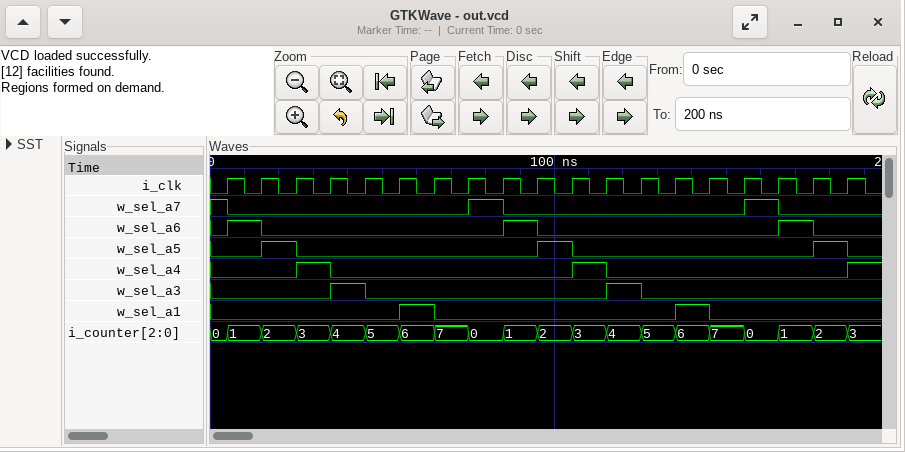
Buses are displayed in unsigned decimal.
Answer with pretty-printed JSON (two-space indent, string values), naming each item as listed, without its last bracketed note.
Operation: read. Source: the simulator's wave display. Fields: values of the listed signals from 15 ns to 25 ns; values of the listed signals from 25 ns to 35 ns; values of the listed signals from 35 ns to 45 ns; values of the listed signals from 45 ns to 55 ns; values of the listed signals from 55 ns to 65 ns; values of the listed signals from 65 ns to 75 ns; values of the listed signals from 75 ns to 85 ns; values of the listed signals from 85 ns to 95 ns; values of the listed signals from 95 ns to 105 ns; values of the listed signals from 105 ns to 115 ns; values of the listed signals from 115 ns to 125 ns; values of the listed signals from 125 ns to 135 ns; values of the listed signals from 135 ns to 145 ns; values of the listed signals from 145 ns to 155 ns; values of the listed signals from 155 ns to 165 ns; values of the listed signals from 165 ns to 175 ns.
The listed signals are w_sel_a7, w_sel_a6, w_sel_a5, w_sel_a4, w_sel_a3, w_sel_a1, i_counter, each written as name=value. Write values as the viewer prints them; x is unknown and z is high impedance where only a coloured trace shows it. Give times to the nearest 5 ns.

{
  "values of the listed signals from 15 ns to 25 ns": "w_sel_a7=0, w_sel_a6=0, w_sel_a5=1, w_sel_a4=0, w_sel_a3=0, w_sel_a1=0, i_counter=2",
  "values of the listed signals from 25 ns to 35 ns": "w_sel_a7=0, w_sel_a6=0, w_sel_a5=0, w_sel_a4=1, w_sel_a3=0, w_sel_a1=0, i_counter=3",
  "values of the listed signals from 35 ns to 45 ns": "w_sel_a7=0, w_sel_a6=0, w_sel_a5=0, w_sel_a4=0, w_sel_a3=1, w_sel_a1=0, i_counter=4",
  "values of the listed signals from 45 ns to 55 ns": "w_sel_a7=0, w_sel_a6=0, w_sel_a5=0, w_sel_a4=0, w_sel_a3=0, w_sel_a1=0, i_counter=5",
  "values of the listed signals from 55 ns to 65 ns": "w_sel_a7=0, w_sel_a6=0, w_sel_a5=0, w_sel_a4=0, w_sel_a3=0, w_sel_a1=1, i_counter=6",
  "values of the listed signals from 65 ns to 75 ns": "w_sel_a7=0, w_sel_a6=0, w_sel_a5=0, w_sel_a4=0, w_sel_a3=0, w_sel_a1=0, i_counter=7",
  "values of the listed signals from 75 ns to 85 ns": "w_sel_a7=1, w_sel_a6=0, w_sel_a5=0, w_sel_a4=0, w_sel_a3=0, w_sel_a1=0, i_counter=0",
  "values of the listed signals from 85 ns to 95 ns": "w_sel_a7=0, w_sel_a6=1, w_sel_a5=0, w_sel_a4=0, w_sel_a3=0, w_sel_a1=0, i_counter=1",
  "values of the listed signals from 95 ns to 105 ns": "w_sel_a7=0, w_sel_a6=0, w_sel_a5=1, w_sel_a4=0, w_sel_a3=0, w_sel_a1=0, i_counter=2",
  "values of the listed signals from 105 ns to 115 ns": "w_sel_a7=0, w_sel_a6=0, w_sel_a5=0, w_sel_a4=1, w_sel_a3=0, w_sel_a1=0, i_counter=3",
  "values of the listed signals from 115 ns to 125 ns": "w_sel_a7=0, w_sel_a6=0, w_sel_a5=0, w_sel_a4=0, w_sel_a3=1, w_sel_a1=0, i_counter=4",
  "values of the listed signals from 125 ns to 135 ns": "w_sel_a7=0, w_sel_a6=0, w_sel_a5=0, w_sel_a4=0, w_sel_a3=0, w_sel_a1=0, i_counter=5",
  "values of the listed signals from 135 ns to 145 ns": "w_sel_a7=0, w_sel_a6=0, w_sel_a5=0, w_sel_a4=0, w_sel_a3=0, w_sel_a1=1, i_counter=6",
  "values of the listed signals from 145 ns to 155 ns": "w_sel_a7=0, w_sel_a6=0, w_sel_a5=0, w_sel_a4=0, w_sel_a3=0, w_sel_a1=0, i_counter=7",
  "values of the listed signals from 155 ns to 165 ns": "w_sel_a7=1, w_sel_a6=0, w_sel_a5=0, w_sel_a4=0, w_sel_a3=0, w_sel_a1=0, i_counter=0",
  "values of the listed signals from 165 ns to 175 ns": "w_sel_a7=0, w_sel_a6=1, w_sel_a5=0, w_sel_a4=0, w_sel_a3=0, w_sel_a1=0, i_counter=1"
}
